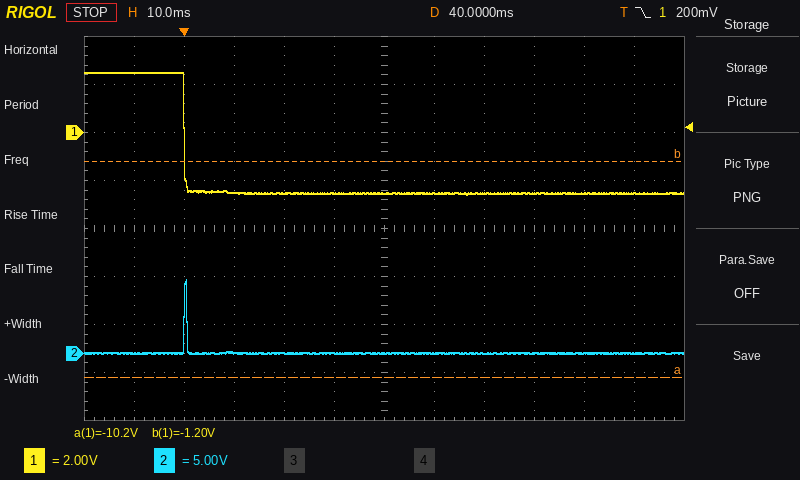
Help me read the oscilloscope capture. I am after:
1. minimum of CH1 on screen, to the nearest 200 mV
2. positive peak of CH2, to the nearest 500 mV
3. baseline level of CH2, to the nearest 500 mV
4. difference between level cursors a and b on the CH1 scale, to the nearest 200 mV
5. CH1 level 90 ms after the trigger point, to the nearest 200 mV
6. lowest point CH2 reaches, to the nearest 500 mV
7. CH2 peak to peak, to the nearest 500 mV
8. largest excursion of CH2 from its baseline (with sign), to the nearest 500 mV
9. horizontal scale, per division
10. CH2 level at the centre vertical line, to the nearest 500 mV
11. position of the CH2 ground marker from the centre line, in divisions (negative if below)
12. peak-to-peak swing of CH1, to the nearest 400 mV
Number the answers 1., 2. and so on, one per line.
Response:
1. -2.6 V
2. 7.5 V
3. 0.0 V
4. 9.0 V
5. -2.6 V
6. 0.0 V
7. 7.5 V
8. +7.5 V
9. 10 ms
10. 0.0 V
11. -2.6 div
12. 5.2 V
